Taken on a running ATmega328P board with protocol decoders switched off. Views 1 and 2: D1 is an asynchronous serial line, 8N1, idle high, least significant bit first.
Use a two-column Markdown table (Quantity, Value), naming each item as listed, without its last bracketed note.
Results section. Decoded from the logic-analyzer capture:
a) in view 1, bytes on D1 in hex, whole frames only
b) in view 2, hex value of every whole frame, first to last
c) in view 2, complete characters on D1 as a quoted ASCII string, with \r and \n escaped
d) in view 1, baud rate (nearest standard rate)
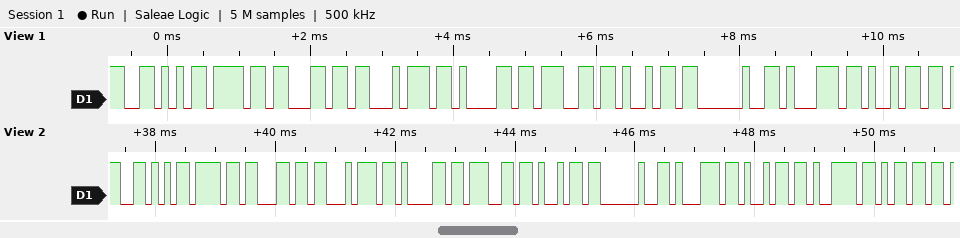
| Quantity | Value |
|---|---|
| in view 1, bytes on D1 in hex, whole frames only | 56 6F 6C 74 61 67 69 20 71 69 |
| in view 2, hex value of every whole frame, first to last | 56 6F 6C 74 61 67 69 20 71 69 79 6D |
| in view 2, complete characters on D1 as a quoted ASCII string, with \r and \n escaped | "Voltagi qiym" |
| in view 1, baud rate | 9600 baud |
